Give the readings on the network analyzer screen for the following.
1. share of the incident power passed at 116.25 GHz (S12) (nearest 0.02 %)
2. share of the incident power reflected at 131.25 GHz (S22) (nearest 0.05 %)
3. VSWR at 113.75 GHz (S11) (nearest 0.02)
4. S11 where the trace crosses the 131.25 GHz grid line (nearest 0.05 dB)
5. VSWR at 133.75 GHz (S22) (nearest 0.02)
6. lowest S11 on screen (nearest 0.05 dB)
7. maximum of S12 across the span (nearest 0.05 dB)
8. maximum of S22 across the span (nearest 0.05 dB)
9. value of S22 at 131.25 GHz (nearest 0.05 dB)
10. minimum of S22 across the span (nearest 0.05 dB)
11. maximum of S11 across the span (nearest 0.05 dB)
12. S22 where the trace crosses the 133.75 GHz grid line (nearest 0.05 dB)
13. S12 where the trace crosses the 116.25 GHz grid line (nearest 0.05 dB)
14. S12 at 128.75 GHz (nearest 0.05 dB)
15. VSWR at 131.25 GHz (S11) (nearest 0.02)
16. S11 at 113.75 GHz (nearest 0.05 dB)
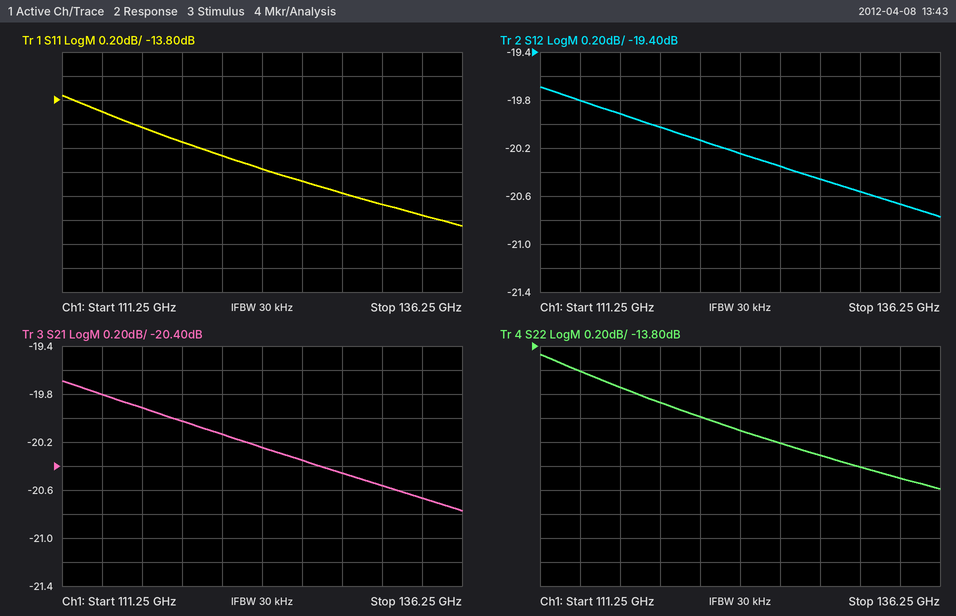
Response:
1.02 %
3.30 %
1.50
-14.65 dB
1.44
-14.85 dB
-19.70 dB
-13.85 dB
-14.80 dB
-15.00 dB
-13.75 dB
-14.90 dB
-19.90 dB
-20.45 dB
1.46
-13.90 dB
